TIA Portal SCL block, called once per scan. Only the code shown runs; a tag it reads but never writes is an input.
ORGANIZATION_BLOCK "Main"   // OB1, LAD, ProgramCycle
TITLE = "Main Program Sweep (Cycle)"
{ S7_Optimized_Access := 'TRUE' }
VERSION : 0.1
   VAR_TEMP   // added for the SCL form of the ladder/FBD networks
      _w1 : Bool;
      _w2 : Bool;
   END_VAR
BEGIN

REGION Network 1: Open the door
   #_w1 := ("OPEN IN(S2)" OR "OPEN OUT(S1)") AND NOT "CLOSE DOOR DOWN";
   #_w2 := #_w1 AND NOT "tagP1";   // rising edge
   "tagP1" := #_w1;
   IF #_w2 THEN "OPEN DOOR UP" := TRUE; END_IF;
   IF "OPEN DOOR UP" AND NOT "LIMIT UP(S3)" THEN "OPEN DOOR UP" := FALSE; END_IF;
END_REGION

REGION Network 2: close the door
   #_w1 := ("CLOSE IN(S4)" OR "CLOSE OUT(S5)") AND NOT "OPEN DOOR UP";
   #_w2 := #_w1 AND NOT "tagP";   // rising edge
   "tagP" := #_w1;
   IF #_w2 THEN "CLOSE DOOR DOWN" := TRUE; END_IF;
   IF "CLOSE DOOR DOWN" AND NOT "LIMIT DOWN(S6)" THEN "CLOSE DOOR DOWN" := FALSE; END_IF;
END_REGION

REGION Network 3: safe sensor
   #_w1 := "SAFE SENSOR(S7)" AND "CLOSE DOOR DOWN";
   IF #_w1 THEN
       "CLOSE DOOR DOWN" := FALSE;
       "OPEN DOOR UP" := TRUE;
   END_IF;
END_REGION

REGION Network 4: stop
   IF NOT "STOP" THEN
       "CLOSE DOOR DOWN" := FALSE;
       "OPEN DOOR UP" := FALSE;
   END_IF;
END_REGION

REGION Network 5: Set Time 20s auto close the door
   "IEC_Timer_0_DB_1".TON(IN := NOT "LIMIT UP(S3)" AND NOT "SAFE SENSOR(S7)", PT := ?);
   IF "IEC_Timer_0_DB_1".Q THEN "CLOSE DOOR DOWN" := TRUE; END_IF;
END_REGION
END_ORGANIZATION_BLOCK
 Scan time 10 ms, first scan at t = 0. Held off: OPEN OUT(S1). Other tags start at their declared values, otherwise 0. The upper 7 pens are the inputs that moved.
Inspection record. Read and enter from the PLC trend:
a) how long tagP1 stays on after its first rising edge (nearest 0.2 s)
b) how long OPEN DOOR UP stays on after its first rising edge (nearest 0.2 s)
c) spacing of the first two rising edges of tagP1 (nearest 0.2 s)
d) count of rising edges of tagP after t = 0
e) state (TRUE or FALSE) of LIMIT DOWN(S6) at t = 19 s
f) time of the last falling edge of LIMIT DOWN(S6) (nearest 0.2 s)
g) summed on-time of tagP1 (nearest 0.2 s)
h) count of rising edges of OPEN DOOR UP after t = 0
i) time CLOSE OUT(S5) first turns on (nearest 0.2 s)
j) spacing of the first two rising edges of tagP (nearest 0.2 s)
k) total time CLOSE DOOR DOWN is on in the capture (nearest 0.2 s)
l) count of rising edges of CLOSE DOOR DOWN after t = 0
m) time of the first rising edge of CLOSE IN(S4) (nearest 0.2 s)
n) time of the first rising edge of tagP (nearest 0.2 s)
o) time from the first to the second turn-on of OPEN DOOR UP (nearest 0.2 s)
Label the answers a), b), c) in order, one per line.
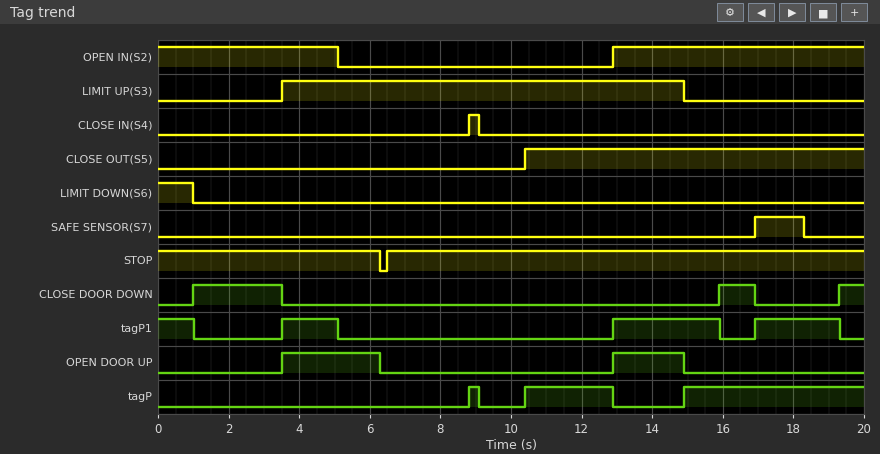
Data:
a) 1.6 s
b) 2.8 s
c) 9.4 s
d) 3
e) FALSE
f) 1.0 s
g) 8.0 s
h) 2
i) 10.4 s
j) 1.6 s
k) 4.2 s
l) 3
m) 8.8 s
n) 8.8 s
o) 9.4 s
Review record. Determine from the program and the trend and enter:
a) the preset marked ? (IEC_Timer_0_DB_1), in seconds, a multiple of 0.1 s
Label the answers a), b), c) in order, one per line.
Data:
a) 1.0 s
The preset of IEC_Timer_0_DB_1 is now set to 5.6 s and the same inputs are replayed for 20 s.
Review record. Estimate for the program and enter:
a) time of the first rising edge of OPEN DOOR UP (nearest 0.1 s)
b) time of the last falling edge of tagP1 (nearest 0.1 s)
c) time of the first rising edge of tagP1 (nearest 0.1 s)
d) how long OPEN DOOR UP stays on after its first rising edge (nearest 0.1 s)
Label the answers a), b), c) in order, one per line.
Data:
a) 12.9 s
b) 5.1 s
c) 12.9 s
d) 2.0 s
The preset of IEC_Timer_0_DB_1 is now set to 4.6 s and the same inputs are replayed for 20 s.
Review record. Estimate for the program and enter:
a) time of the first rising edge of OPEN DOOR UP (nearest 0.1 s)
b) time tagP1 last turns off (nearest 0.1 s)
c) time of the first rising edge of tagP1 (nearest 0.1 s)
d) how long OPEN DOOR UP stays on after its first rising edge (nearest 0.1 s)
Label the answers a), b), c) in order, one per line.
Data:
a) 12.9 s
b) 5.1 s
c) 12.9 s
d) 2.0 s
